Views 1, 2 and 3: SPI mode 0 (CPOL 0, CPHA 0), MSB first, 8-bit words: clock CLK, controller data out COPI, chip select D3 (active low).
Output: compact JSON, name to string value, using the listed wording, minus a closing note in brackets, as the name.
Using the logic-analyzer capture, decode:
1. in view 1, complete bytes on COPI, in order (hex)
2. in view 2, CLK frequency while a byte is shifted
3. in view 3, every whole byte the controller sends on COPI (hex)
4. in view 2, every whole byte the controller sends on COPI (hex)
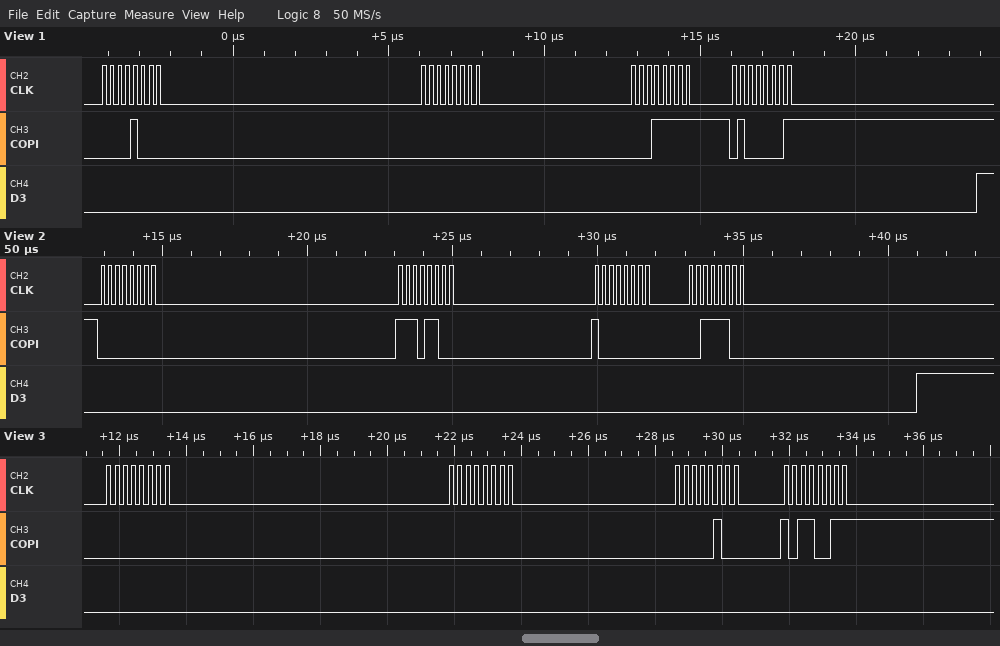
{"in view 1, complete bytes on COPI, in order": "08 00 1F 41", "in view 2, CLK frequency while a byte is shifted": "4 MHz", "in view 3, every whole byte the controller sends on COPI": "00 00 04 B3", "in view 2, every whole byte the controller sends on COPI": "00 EC 80 3C"}
